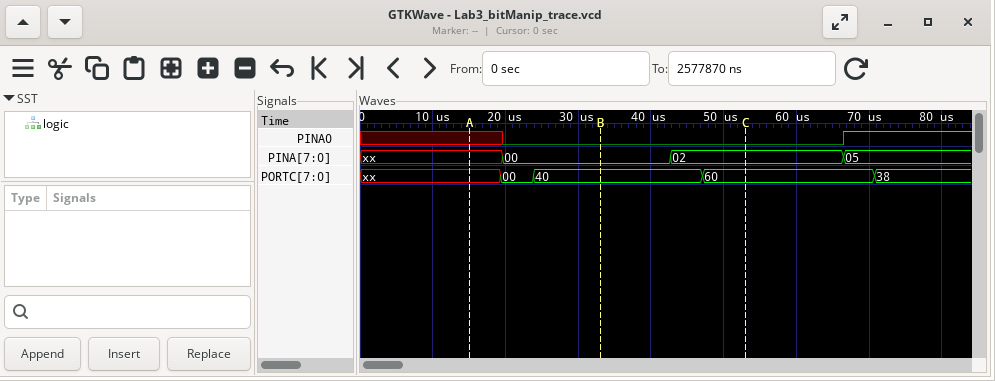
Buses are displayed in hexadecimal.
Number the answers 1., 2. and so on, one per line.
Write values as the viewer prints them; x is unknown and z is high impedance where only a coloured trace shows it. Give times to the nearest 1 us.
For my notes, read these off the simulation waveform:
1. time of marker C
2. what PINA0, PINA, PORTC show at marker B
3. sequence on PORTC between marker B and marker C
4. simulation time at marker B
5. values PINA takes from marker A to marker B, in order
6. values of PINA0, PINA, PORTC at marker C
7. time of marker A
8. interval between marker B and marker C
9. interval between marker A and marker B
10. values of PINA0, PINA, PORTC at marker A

1. 53 us
2. PINA0=0, PINA=00, PORTC=40
3. 40, 60
4. 33 us
5. xx, 00
6. PINA0=0, PINA=02, PORTC=60
7. 15 us
8. 20 us
9. 18 us
10. PINA0=x, PINA=xx, PORTC=xx
